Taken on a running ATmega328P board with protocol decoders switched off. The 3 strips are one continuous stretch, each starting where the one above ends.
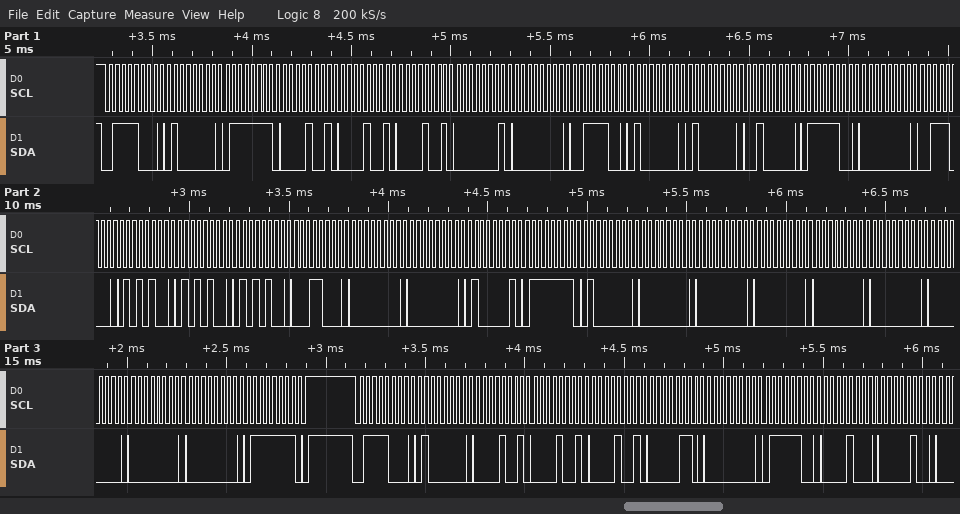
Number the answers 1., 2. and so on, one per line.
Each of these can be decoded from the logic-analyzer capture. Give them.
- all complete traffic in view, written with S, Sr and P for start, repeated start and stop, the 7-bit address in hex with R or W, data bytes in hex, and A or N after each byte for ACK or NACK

1. S 3CW A 40 A 7F A 09 A 09 A 09 A 01 A 00 A 3C A 40 A 40 A 20 A 7C A 00 A 38 A 54 A 54 A 54 A 18 A 00 A 00 A 41 A 7F A 40 A 00 A 00 A 00 A 00 A 00 A 00 A 00 A 00 A 7F A P S 3CW A 40 A 09 A 09 A 09 A 06 A 00 A 7C A 08 A 04 A
